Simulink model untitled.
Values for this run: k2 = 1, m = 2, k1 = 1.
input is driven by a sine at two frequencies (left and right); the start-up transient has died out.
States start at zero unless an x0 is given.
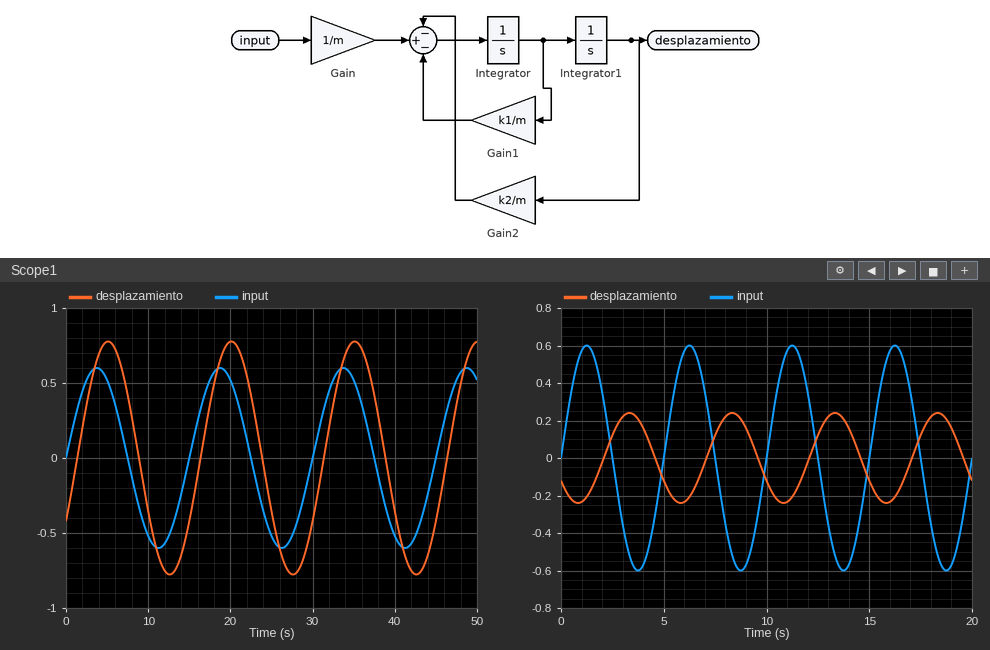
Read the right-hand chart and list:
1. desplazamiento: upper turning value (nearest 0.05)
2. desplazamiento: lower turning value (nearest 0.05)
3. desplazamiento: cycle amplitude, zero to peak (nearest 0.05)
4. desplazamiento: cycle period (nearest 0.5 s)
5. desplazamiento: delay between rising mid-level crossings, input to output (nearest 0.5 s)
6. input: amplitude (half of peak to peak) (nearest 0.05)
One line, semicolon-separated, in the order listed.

0.25; -0.25; 0.25; 5.0 s; 2.0 s; 0.60
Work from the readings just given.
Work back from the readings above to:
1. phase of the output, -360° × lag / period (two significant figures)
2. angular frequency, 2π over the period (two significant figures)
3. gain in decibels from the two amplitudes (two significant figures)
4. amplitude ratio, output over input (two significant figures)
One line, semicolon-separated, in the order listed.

-140°; 1.3 rad/s; -7.6 dB; 0.42
